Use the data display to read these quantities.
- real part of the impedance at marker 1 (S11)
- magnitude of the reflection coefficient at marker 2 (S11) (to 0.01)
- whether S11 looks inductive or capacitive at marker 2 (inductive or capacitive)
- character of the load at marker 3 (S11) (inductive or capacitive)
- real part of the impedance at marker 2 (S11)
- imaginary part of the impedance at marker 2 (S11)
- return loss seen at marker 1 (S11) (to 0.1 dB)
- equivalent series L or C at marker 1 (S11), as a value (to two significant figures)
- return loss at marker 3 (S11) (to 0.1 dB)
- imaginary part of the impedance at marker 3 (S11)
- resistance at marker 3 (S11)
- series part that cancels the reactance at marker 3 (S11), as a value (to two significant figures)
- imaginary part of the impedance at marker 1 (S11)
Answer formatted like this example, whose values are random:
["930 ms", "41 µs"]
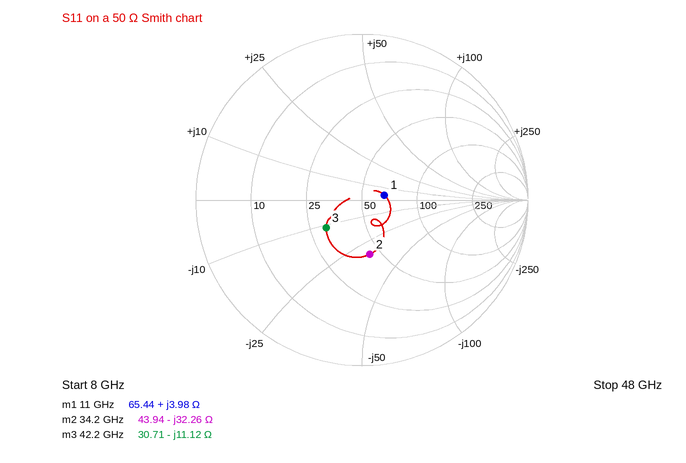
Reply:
["65.44 Ω", "0.33", "capacitive", "capacitive", "43.94 Ω", "-32.26 Ω", "17.2 dB", "58 pH", "11.3 dB", "-11.12 Ω", "30.71 Ω", "42 pH", "+3.98 Ω"]
